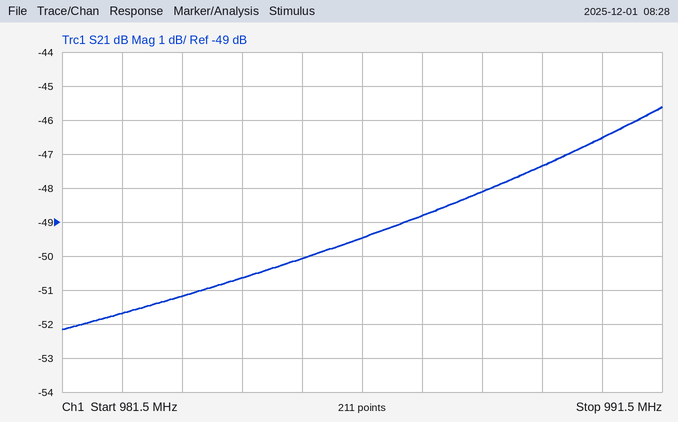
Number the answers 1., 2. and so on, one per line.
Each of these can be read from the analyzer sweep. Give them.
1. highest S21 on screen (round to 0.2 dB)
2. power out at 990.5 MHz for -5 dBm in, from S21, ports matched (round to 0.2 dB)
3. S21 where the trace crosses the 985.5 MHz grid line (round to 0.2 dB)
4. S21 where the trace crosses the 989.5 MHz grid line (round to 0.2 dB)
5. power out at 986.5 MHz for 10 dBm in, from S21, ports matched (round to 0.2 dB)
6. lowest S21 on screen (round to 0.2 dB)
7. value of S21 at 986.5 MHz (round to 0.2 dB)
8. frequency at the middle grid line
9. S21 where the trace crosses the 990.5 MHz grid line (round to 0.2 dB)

1. -45.6 dB
2. -51.6 dBm
3. -50.0 dB
4. -47.4 dB
5. -39.4 dBm
6. -52.2 dB
7. -49.4 dB
8. 986.5 MHz
9. -46.6 dB
